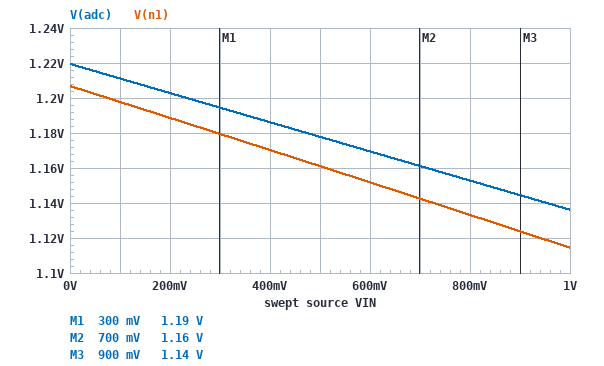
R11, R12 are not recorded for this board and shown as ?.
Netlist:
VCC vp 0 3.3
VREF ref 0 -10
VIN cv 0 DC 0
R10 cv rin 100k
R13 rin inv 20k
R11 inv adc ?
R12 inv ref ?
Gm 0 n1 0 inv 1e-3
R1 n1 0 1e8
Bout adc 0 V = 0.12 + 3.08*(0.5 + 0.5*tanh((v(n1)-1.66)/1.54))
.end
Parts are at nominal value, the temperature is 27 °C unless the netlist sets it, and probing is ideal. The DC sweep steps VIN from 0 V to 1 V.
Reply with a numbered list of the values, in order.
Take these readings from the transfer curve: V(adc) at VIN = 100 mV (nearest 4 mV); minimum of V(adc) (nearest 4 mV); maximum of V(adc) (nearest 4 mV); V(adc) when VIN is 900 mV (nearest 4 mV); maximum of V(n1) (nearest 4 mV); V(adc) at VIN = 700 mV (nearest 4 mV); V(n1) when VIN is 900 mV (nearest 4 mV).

1. 1.212 V
2. 1.136 V
3. 1.220 V
4. 1.144 V
5. 1.208 V
6. 1.160 V
7. 1.124 V
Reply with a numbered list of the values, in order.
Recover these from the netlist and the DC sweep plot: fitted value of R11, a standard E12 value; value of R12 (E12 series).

1. 10 kΩ
2. 82 kΩ
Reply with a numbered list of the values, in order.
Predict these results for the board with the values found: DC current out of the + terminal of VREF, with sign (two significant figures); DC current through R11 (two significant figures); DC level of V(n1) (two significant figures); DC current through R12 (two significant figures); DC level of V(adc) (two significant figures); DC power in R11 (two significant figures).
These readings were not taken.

1. -120 µA
2. 120 µA
3. 1.2 V
4. 120 µA
5. 1.2 V
6. 150 µW
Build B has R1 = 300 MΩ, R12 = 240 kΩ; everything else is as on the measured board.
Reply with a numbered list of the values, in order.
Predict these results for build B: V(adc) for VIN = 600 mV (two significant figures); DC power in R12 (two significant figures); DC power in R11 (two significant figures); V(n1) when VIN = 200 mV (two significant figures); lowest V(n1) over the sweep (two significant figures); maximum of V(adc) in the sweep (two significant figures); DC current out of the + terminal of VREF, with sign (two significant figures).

1. 370 mV
2. 420 µW
3. 17 µW
4. -110 mV
5. -340 mV
6. 420 mV
7. -42 µA
